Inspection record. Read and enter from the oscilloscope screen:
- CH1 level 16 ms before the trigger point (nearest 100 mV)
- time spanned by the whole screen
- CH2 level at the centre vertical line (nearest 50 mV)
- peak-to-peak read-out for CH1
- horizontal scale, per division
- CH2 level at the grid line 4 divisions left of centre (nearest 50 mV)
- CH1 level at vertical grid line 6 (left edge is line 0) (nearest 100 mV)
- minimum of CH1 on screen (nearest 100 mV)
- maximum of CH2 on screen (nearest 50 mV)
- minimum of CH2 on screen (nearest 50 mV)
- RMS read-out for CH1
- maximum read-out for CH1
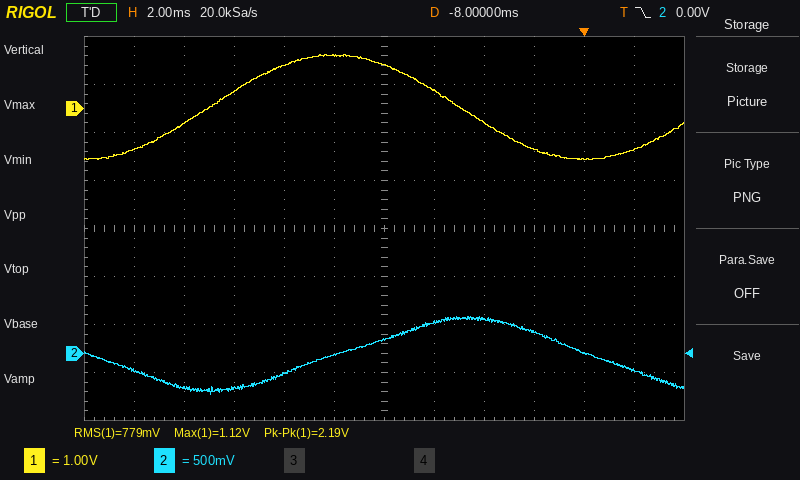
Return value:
-300 mV
24 ms
150 mV
2.19 V
2 ms
-350 mV
900 mV
-1.1 V
400 mV
-450 mV
779 mV
1.12 V
